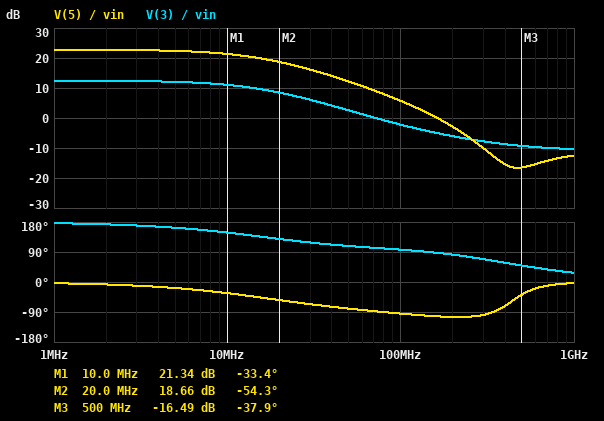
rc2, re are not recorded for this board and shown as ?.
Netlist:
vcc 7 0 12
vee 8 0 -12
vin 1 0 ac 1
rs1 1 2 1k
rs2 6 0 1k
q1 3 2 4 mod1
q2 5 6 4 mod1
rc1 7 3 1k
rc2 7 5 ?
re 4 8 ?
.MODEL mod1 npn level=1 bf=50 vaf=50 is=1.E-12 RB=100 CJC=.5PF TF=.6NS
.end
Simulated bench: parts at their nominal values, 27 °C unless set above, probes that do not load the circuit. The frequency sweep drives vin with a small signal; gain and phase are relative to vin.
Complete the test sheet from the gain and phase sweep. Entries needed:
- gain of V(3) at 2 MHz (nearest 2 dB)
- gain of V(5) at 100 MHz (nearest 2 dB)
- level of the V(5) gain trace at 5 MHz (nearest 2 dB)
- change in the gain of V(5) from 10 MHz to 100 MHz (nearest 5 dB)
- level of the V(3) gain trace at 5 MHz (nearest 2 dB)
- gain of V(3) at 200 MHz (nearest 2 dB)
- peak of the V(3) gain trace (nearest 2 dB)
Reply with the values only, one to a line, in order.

12 dB
6 dB
22 dB
-15 dB
12 dB
-6 dB
12 dB
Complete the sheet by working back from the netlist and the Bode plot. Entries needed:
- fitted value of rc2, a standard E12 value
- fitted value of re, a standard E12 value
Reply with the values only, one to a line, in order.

3.3 kΩ
22 kΩ
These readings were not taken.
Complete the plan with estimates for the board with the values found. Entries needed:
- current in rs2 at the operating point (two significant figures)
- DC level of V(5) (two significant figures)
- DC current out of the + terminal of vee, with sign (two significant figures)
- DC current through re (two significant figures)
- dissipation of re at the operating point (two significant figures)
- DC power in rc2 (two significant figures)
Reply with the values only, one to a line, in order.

4.2 µA
11 V
-520 µA
520 µA
6.0 mW
220 µW
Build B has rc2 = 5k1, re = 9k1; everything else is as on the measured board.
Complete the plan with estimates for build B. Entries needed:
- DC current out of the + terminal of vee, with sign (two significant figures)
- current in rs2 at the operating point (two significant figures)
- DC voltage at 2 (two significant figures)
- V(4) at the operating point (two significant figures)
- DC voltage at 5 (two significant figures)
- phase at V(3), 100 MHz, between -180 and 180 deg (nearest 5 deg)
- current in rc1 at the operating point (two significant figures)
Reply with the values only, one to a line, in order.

-1.3 mA
10 µA
-10 mV
-530 mV
8.9 V
100 deg
630 µA
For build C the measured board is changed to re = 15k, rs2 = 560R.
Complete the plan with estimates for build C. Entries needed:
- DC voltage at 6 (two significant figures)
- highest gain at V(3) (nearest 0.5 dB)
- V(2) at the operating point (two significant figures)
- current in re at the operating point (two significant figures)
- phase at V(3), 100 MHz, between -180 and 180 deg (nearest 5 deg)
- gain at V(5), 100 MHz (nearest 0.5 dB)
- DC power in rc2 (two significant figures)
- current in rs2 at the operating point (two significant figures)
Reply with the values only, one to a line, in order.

-3.6 mV
15.5 dB
-5.9 mV
770 µA
95 deg
8.5 dB
500 µW
6.4 µA
